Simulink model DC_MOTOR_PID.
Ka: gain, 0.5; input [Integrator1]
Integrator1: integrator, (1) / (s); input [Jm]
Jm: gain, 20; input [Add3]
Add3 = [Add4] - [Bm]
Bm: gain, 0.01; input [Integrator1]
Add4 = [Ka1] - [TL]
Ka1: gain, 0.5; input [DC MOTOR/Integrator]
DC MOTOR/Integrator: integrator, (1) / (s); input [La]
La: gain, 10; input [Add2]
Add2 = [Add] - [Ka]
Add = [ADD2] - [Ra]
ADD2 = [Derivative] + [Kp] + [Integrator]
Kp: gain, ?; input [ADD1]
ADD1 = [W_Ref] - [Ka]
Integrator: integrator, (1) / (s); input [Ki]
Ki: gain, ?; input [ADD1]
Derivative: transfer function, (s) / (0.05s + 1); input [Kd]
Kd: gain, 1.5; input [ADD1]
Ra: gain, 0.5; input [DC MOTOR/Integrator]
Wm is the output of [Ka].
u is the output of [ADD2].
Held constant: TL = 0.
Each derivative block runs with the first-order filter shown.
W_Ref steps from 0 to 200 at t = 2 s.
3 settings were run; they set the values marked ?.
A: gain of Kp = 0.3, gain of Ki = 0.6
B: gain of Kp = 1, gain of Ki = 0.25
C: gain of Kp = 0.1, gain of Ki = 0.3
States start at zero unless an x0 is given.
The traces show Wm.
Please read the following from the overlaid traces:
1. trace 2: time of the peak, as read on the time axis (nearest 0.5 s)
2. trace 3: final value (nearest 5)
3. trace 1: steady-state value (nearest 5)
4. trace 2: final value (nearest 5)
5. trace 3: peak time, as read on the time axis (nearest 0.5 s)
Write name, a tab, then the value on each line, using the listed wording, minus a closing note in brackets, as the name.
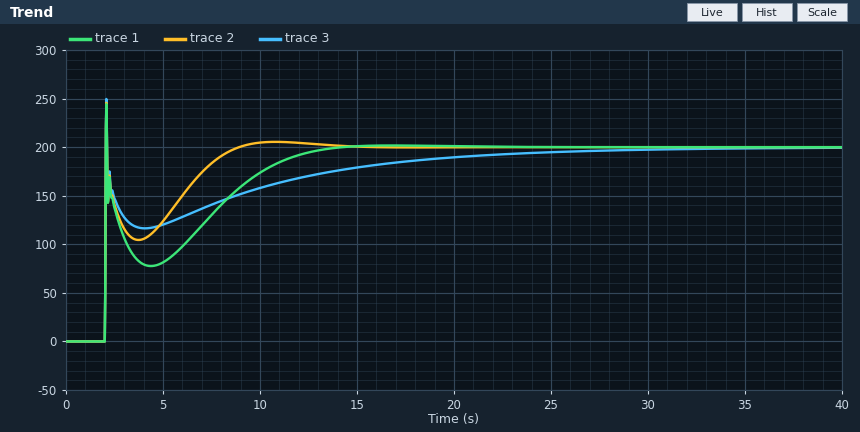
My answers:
trace 2: time of the peak, as read on the time axis	2.0 s
trace 3: final value	200
trace 1: steady-state value	200
trace 2: final value	200
trace 3: peak time, as read on the time axis	2.0 s
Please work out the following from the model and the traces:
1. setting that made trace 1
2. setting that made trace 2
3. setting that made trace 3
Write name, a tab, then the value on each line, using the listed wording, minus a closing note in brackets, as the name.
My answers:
setting that made trace 1	C
setting that made trace 2	A
setting that made trace 3	B
